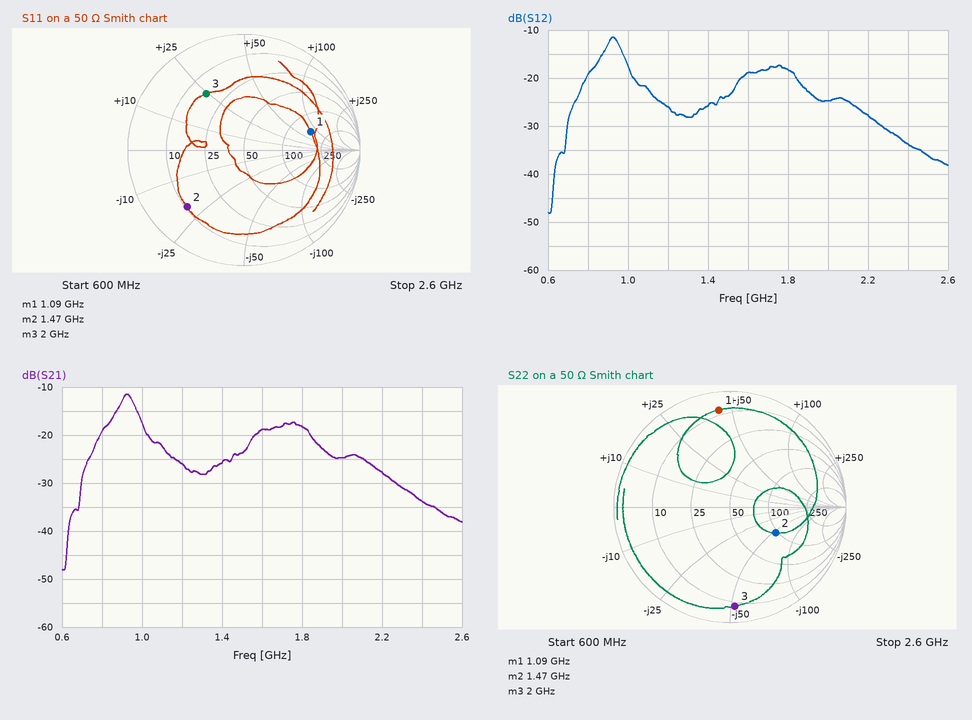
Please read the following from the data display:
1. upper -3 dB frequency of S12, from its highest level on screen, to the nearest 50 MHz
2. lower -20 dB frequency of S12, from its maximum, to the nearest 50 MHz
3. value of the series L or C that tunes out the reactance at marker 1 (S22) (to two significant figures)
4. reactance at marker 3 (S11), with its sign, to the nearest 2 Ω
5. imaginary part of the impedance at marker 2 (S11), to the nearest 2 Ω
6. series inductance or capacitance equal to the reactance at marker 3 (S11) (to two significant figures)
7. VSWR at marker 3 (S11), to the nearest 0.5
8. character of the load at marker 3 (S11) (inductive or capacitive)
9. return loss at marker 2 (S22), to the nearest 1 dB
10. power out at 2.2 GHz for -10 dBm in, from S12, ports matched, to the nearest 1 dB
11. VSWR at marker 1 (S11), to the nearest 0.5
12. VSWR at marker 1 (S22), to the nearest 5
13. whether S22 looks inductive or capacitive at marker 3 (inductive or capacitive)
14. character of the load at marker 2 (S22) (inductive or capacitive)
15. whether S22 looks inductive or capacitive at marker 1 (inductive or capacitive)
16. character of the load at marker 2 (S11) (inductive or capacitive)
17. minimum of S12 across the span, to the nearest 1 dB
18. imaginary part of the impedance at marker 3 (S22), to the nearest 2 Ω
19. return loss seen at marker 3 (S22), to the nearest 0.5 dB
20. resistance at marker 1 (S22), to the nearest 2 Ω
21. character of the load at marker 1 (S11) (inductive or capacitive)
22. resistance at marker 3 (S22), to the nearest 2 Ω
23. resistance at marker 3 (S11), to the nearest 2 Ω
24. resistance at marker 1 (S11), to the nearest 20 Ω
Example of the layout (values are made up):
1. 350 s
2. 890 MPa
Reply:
1. 950 MHz
2. 700 MHz
3. 3.3 pF
4. +24 Ω
5. -20 Ω
6. 1.9 nH
7. 4.0
8. inductive
9. 7 dB
10. -38 dBm
11. 4.0
12. 10
13. capacitive
14. capacitive
15. inductive
16. capacitive
17. -48 dB
18. -52 Ω
19. 1.5 dB
20. 8 Ω
21. inductive
22. 8 Ω
23. 16 Ω
24. 160 Ω
